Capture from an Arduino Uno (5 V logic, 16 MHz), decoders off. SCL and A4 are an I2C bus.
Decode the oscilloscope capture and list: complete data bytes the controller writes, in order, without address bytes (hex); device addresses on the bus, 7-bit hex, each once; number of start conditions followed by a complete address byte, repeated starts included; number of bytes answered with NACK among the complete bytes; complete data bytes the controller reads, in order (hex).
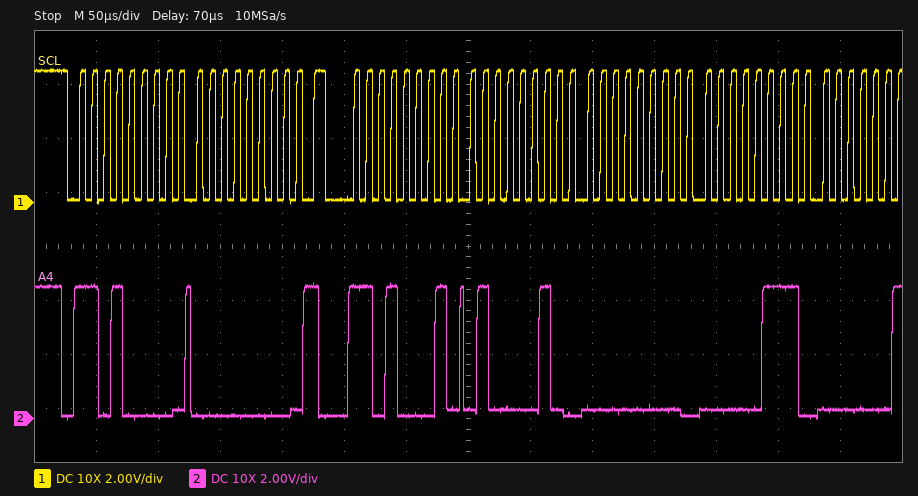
00
0x68
2
0
42 00 07
